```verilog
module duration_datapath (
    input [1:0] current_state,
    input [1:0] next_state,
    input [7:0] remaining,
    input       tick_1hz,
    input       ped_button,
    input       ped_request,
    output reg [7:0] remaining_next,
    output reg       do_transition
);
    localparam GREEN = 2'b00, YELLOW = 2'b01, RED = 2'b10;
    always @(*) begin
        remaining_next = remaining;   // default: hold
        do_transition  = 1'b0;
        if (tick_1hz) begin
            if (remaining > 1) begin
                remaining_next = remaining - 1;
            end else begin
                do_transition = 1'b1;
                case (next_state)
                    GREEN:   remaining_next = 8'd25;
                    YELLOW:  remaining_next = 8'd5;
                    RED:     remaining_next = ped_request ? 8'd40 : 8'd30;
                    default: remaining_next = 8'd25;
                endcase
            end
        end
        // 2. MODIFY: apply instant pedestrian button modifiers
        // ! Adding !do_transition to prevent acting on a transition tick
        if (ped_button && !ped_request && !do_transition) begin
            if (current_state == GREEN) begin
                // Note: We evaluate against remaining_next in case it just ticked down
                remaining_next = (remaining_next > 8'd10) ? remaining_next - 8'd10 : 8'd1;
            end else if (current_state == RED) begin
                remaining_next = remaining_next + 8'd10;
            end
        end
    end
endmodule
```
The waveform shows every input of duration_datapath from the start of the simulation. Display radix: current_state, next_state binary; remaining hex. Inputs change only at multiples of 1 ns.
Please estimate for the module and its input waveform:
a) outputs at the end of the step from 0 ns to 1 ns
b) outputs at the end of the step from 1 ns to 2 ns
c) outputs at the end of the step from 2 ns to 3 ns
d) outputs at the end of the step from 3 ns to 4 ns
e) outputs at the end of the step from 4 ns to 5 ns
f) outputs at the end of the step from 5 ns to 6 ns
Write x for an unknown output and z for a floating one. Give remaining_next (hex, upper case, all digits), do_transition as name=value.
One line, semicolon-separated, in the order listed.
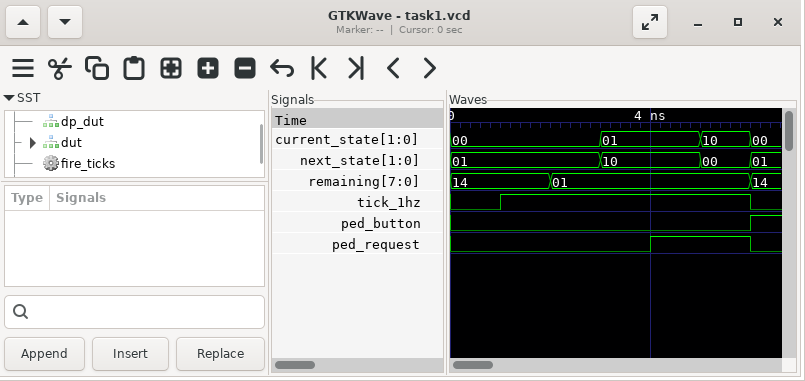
remaining_next=14, do_transition=0; remaining_next=13, do_transition=0; remaining_next=05, do_transition=1; remaining_next=1E, do_transition=1; remaining_next=28, do_transition=1; remaining_next=19, do_transition=1
